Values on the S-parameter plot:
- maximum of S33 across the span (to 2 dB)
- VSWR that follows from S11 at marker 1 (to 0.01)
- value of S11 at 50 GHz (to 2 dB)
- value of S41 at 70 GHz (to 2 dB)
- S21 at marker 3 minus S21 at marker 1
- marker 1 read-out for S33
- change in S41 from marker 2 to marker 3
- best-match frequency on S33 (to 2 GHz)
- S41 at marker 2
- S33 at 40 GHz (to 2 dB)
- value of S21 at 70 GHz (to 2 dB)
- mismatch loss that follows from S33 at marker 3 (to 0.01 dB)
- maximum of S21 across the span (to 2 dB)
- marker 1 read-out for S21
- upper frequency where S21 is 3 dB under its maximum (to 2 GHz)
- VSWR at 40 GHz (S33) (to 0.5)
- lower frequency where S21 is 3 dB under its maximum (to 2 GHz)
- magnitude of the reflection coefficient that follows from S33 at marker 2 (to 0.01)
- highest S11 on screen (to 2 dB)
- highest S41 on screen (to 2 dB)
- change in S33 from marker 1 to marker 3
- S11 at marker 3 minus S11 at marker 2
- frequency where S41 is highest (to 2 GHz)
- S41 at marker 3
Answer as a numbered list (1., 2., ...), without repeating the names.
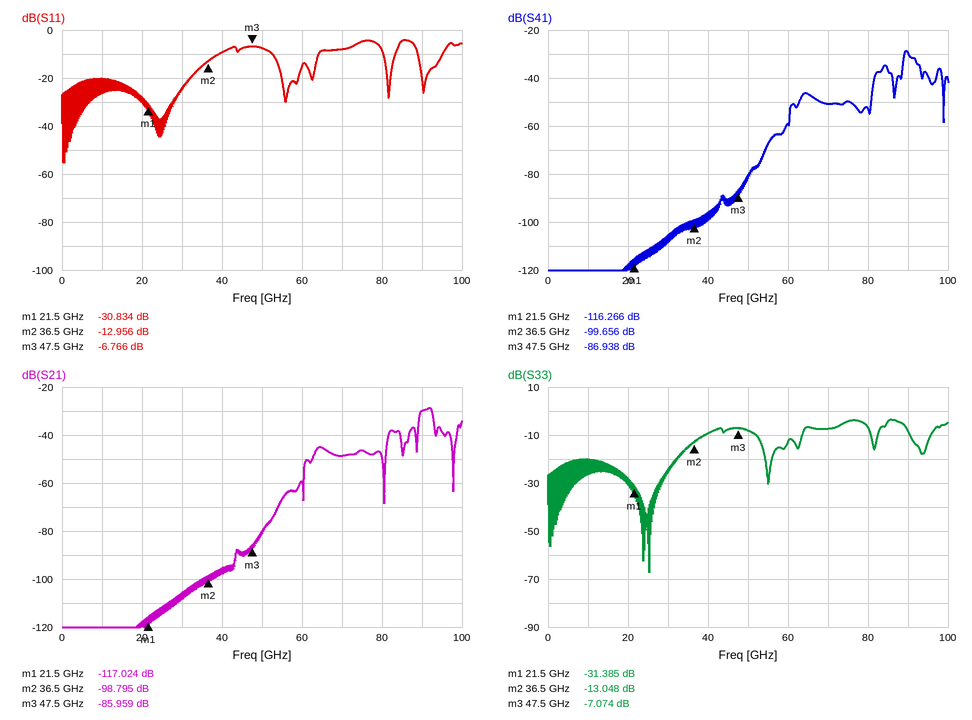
1. -4 dB
2. 1.06
3. -8 dB
4. -50 dB
5. 31.065 dB
6. -31.385 dB
7. 12.718 dB
8. 26 GHz
9. -99.656 dB
10. -10 dB
11. -48 dB
12. 0.95 dB
13. -28 dB
14. -117.024 dB
15. 92 GHz
16. 2.0
17. 90 GHz
18. 0.22
19. -4 dB
20. -28 dB
21. 24.311 dB
22. 6.190 dB
23. 90 GHz
24. -86.938 dB
